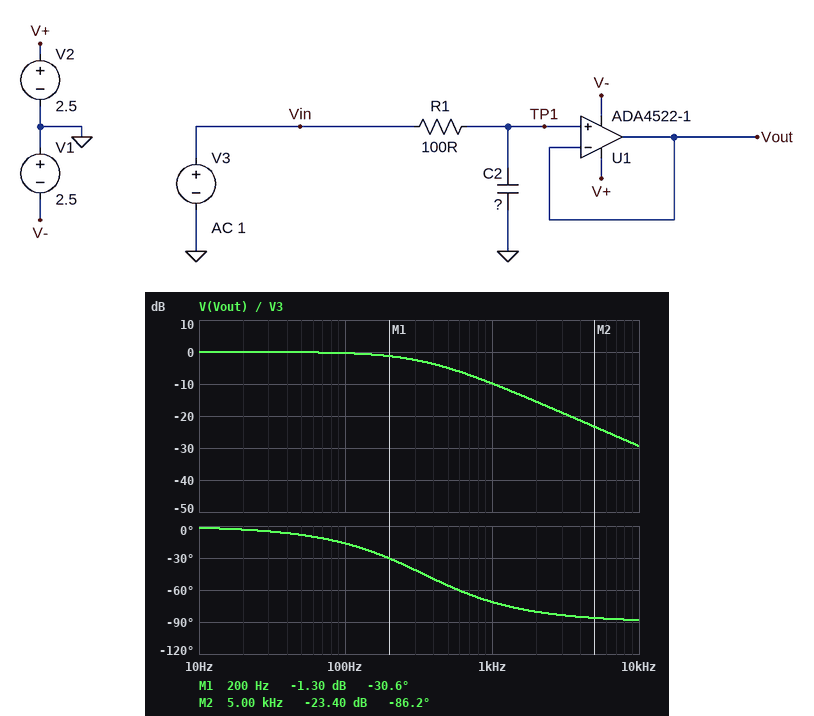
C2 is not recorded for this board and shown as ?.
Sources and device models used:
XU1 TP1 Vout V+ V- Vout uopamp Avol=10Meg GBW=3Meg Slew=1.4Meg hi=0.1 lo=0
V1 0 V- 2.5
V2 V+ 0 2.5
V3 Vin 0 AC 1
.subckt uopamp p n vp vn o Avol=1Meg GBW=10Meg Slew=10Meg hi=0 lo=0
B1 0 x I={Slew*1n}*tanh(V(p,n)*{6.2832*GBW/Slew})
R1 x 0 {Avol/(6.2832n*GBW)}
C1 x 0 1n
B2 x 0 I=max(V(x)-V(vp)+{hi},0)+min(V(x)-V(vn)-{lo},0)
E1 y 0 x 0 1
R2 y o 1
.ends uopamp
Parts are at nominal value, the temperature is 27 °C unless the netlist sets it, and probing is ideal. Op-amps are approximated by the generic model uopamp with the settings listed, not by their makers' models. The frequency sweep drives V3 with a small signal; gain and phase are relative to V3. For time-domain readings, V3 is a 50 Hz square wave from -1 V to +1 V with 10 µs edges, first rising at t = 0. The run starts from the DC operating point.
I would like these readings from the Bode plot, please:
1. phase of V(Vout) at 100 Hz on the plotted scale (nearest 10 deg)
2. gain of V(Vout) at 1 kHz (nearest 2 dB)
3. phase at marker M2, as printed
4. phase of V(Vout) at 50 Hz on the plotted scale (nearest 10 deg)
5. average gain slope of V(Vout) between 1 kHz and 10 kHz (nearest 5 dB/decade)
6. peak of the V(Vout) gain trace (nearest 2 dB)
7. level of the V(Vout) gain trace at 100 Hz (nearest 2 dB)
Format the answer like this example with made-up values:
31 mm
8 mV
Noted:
-20 deg
-10 dB
-86.2 deg
-10 deg
-20 dB/decade
0 dB
0 dB
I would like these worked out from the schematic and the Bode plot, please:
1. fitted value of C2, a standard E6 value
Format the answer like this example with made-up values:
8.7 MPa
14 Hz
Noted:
4.7 µF
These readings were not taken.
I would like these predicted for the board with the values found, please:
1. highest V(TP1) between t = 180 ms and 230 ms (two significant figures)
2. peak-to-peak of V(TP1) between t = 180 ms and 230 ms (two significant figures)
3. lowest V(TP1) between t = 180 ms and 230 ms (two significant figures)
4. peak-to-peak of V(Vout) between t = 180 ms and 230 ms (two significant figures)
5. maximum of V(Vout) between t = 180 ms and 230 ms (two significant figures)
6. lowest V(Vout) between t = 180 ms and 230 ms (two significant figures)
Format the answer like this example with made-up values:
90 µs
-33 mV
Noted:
1.0 V
2.0 V
-1.0 V
2.0 V
1.0 V
-1.0 V
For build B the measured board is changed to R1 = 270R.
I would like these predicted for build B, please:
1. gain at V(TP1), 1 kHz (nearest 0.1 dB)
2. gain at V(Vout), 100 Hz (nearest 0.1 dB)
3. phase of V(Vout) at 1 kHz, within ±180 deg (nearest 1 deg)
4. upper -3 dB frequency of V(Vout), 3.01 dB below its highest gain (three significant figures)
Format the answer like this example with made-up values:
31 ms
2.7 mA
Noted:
-18.1 dB
-2.1 dB
-83 deg
125 Hz
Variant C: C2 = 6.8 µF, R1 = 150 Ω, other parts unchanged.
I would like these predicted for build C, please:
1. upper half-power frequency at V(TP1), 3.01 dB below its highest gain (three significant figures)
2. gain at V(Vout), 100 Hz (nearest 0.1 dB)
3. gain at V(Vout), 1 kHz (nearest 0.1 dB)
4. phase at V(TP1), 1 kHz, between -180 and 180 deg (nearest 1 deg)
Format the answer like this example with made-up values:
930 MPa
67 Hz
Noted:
156 Hz
-1.5 dB
-16.2 dB
-81 deg
